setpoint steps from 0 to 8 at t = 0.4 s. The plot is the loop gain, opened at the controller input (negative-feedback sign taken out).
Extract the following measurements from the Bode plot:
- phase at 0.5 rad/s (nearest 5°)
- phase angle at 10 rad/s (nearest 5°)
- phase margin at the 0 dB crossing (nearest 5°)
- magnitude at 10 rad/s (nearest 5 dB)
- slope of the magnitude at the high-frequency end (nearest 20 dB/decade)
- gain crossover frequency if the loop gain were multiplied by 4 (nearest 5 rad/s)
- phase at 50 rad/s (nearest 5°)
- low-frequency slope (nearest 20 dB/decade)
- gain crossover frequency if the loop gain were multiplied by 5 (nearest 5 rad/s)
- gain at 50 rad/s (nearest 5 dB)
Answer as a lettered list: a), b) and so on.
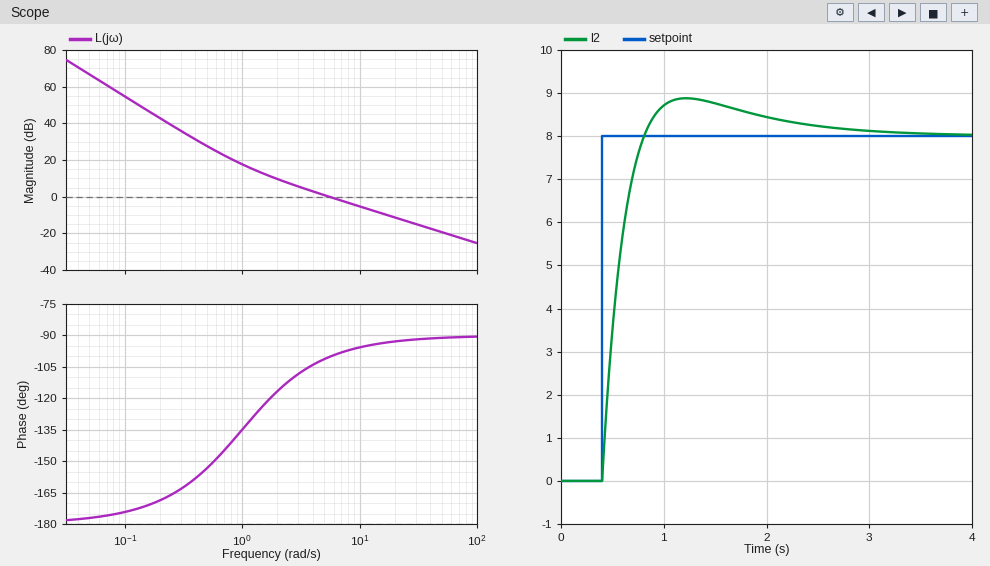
a) -155°
b) -95°
c) 80°
d) -5 dB
e) -20 dB/decade
f) 20 rad/s
g) -90°
h) -40 dB/decade
i) 25 rad/s
j) -20 dB
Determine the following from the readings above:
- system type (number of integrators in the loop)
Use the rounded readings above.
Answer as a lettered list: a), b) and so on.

a) 2
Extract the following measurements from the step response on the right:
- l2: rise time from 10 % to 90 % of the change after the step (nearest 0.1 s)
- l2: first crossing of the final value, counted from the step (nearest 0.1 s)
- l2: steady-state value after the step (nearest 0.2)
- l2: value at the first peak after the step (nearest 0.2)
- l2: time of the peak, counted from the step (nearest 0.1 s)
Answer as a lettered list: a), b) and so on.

a) 0.3 s
b) 0.4 s
c) 8.0
d) 8.8
e) 0.8 s
